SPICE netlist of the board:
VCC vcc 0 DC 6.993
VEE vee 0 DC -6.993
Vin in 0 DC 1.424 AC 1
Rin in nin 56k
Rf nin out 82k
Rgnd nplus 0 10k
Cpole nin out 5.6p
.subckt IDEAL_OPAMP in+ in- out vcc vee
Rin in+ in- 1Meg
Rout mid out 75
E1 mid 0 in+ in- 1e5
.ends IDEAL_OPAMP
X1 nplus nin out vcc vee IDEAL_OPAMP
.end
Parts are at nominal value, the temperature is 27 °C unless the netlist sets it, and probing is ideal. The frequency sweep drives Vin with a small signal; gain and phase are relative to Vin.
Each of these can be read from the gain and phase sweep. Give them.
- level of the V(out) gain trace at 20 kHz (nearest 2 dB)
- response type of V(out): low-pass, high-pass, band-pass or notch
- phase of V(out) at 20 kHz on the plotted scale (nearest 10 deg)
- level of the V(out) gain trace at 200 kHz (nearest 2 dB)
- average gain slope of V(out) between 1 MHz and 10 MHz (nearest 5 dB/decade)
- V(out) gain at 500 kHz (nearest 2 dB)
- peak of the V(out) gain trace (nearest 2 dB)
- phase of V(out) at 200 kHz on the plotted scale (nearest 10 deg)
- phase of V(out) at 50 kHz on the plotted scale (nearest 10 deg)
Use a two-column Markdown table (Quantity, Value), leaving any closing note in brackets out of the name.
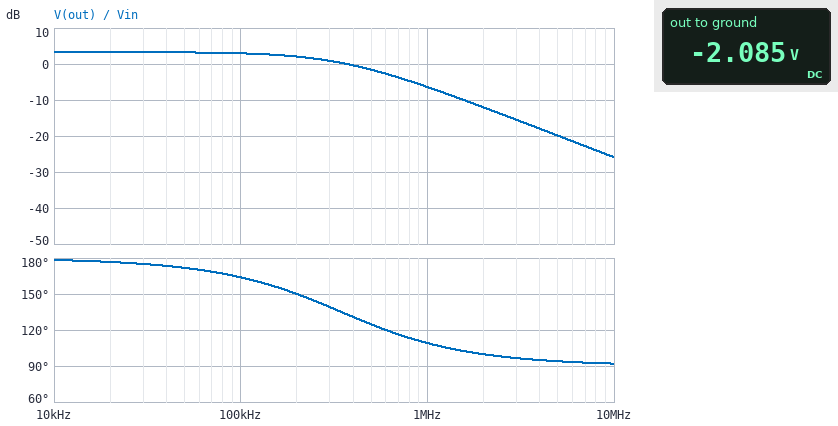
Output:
| Quantity | Value |
|---|---|
| level of the V(out) gain trace at 20 kHz | 4 dB |
| response type of V(out): low-pass, high-pass, band-pass or notch | low-pass |
| phase of V(out) at 20 kHz on the plotted scale | 180 deg |
| level of the V(out) gain trace at 200 kHz | 2 dB |
| average gain slope of V(out) between 1 MHz and 10 MHz | -20 dB/decade |
| V(out) gain at 500 kHz | -2 dB |
| peak of the V(out) gain trace | 4 dB |
| phase of V(out) at 200 kHz on the plotted scale | 150 deg |
| phase of V(out) at 50 kHz on the plotted scale | 170 deg |
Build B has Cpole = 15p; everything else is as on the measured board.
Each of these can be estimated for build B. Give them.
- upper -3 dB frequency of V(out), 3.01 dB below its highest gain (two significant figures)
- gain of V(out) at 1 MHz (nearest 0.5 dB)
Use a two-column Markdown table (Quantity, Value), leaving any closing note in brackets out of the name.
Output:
| Quantity | Value |
|---|---|
| upper -3 dB frequency of V(out), 3.01 dB below its highest gain | 130 kHz |
| gain of V(out) at 1 MHz | -14.5 dB |
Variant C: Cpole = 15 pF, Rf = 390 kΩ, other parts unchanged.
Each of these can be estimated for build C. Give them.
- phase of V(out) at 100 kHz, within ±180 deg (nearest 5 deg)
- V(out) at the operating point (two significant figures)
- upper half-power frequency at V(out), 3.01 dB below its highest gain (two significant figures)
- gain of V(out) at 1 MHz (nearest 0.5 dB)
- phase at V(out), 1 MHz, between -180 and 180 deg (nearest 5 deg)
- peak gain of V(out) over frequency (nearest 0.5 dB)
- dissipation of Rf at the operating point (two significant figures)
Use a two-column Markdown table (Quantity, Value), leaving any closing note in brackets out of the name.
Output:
| Quantity | Value |
|---|---|
| phase of V(out) at 100 kHz, within ±180 deg | 105 deg |
| V(out) at the operating point | -9.9 V |
| upper half-power frequency at V(out), 3.01 dB below its highest gain | 27 kHz |
| gain of V(out) at 1 MHz | -14.5 dB |
| phase at V(out), 1 MHz, between -180 and 180 deg | 90 deg |
| peak gain of V(out) over frequency | 17.0 dB |
| dissipation of Rf at the operating point | 250 µW |
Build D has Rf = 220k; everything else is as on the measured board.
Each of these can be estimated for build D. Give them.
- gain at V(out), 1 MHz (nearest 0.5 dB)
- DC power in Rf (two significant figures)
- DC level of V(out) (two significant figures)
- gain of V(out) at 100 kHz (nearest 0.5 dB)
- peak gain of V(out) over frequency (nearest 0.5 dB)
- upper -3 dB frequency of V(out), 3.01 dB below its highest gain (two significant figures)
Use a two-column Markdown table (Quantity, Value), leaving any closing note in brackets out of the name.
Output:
| Quantity | Value |
|---|---|
| gain at V(out), 1 MHz | -6.0 dB |
| DC power in Rf | 140 µW |
| DC level of V(out) | -5.6 V |
| gain of V(out) at 100 kHz | 10.0 dB |
| peak gain of V(out) over frequency | 12.0 dB |
| upper -3 dB frequency of V(out), 3.01 dB below its highest gain | 130 kHz |
